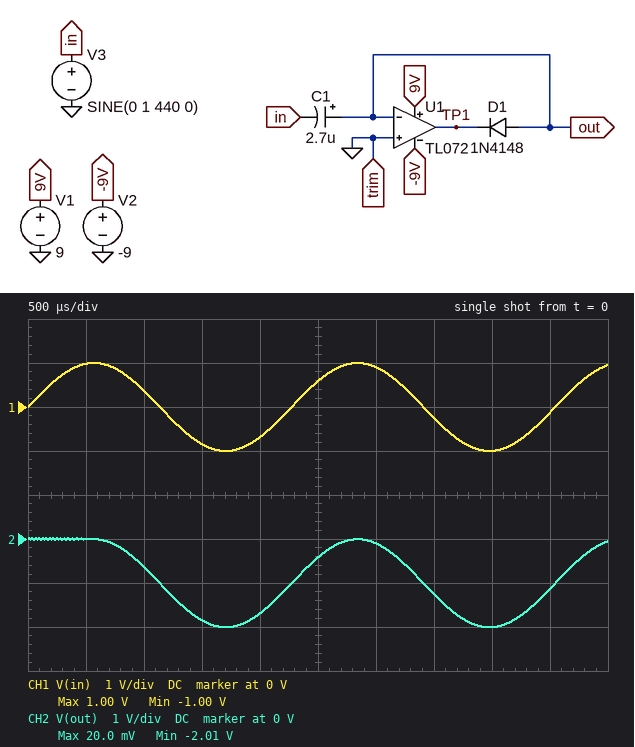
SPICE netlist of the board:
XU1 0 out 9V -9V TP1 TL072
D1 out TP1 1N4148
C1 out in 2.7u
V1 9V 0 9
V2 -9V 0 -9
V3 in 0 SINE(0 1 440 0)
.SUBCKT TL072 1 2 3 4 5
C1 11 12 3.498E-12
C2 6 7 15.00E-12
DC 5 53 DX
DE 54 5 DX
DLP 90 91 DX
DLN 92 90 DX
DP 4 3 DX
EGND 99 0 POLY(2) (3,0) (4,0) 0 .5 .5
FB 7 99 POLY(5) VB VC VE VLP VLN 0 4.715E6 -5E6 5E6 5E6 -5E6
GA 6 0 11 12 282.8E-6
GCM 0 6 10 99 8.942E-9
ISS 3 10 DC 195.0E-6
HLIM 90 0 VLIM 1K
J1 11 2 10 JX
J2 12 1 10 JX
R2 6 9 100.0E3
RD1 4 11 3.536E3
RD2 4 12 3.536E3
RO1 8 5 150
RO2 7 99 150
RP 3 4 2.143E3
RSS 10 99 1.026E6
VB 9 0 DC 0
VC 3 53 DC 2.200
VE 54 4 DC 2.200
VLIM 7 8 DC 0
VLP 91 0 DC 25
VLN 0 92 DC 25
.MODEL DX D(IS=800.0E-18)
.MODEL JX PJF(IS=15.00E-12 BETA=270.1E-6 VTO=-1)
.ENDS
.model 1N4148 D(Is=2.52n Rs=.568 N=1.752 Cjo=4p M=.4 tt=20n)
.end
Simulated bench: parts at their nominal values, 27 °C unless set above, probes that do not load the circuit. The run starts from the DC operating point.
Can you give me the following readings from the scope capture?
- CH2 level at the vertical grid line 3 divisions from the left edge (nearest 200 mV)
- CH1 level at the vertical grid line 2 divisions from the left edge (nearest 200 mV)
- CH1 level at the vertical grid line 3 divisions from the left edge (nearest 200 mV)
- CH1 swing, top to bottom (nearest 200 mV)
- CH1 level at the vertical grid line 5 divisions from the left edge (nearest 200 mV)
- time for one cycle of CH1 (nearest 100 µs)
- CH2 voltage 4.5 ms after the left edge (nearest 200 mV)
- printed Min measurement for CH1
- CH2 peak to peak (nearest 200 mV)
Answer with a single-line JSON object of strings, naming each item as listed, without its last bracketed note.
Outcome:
{"CH2 level at the vertical grid line 3 divisions from the left edge": "-1.8 V", "CH1 level at the vertical grid line 2 divisions from the left edge": "400 mV", "CH1 level at the vertical grid line 3 divisions from the left edge": "-800 mV", "CH1 swing, top to bottom": "2.0 V", "CH1 level at the vertical grid line 5 divisions from the left edge": "600 mV", "time for one cycle of CH1": "2.3 ms", "CH2 voltage 4.5 ms after the left edge": "-1.2 V", "printed Min measurement for CH1": "-1.00 V", "CH2 peak to peak": "2.0 V"}
